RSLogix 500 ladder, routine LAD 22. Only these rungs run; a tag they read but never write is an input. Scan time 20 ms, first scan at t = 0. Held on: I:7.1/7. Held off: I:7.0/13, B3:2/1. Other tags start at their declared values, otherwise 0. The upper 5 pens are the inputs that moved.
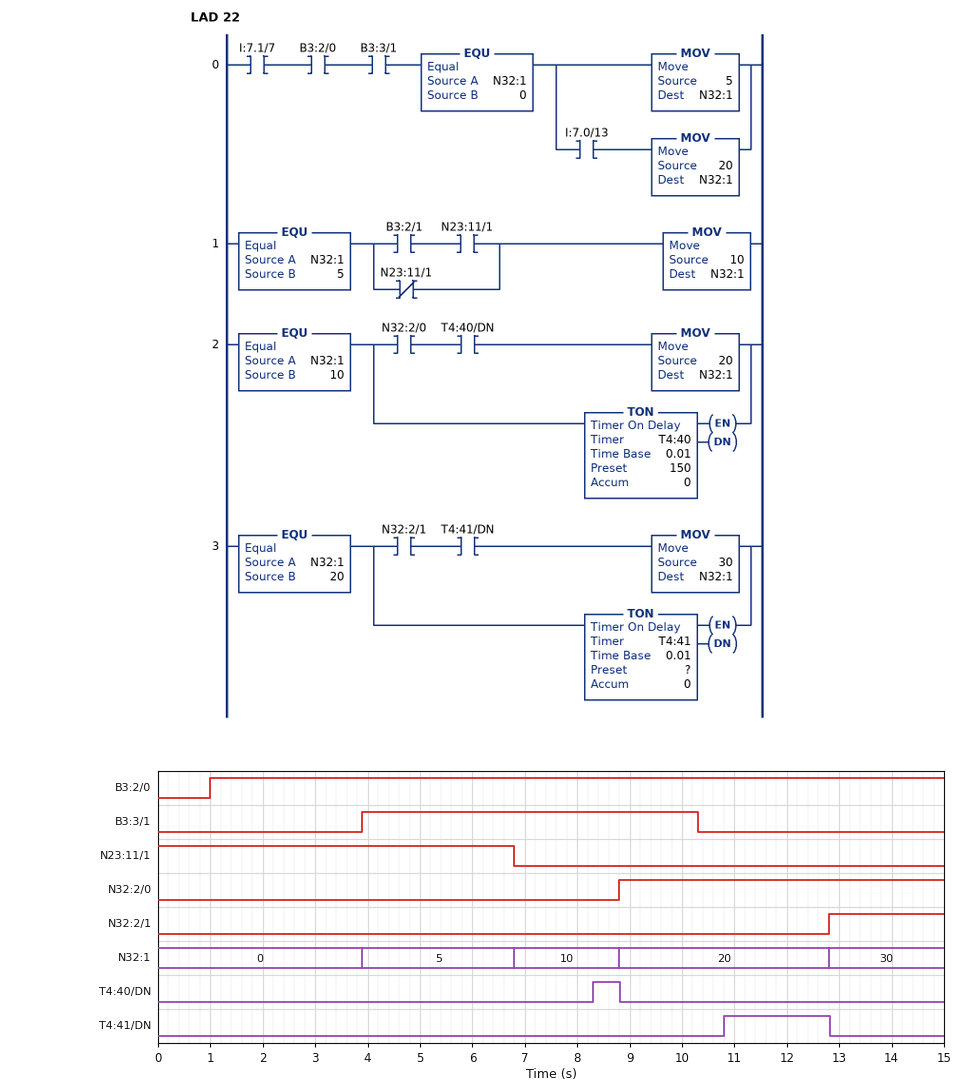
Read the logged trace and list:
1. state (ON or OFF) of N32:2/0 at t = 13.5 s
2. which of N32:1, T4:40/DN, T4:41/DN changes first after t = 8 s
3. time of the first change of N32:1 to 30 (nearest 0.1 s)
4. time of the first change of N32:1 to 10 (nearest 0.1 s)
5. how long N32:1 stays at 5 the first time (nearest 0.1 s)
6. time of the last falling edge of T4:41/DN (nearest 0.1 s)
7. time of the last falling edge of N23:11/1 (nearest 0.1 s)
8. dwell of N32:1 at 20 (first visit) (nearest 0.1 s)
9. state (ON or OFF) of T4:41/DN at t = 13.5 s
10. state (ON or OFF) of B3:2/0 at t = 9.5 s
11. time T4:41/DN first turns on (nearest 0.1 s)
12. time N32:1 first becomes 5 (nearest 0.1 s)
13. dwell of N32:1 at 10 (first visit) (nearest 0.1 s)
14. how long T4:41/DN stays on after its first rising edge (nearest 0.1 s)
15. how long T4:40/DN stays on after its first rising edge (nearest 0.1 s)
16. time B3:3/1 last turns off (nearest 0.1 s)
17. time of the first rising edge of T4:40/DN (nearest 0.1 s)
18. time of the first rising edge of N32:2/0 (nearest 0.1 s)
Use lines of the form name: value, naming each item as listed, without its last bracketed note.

state (ON or OFF) of N32:2/0 at t = 13.5 s: ON
which of N32:1, T4:40/DN, T4:41/DN changes first after t = 8 s: T4:40/DN
time of the first change of N32:1 to 30: 12.8 s
time of the first change of N32:1 to 10: 6.8 s
how long N32:1 stays at 5 the first time: 2.9 s
time of the last falling edge of T4:41/DN: 12.8 s
time of the last falling edge of N23:11/1: 6.8 s
dwell of N32:1 at 20 (first visit): 4.0 s
state (ON or OFF) of T4:41/DN at t = 13.5 s: OFF
state (ON or OFF) of B3:2/0 at t = 9.5 s: ON
time T4:41/DN first turns on: 10.8 s
time N32:1 first becomes 5: 3.9 s
dwell of N32:1 at 10 (first visit): 2.0 s
how long T4:41/DN stays on after its first rising edge: 2.0 s
how long T4:40/DN stays on after its first rising edge: 0.5 s
time B3:3/1 last turns off: 10.3 s
time of the first rising edge of T4:40/DN: 8.3 s
time of the first rising edge of N32:2/0: 8.8 s
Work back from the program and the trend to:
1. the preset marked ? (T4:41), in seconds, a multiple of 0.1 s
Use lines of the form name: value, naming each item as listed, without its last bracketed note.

the preset marked ? (T4:41), in seconds, a multiple of 0.1 s: 2.0 s
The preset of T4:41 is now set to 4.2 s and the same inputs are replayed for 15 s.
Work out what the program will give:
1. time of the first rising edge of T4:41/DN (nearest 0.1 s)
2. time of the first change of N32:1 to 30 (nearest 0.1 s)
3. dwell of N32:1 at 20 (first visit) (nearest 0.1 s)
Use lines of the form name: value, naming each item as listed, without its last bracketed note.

time of the first rising edge of T4:41/DN: 13.0 s
time of the first change of N32:1 to 30: 13.0 s
dwell of N32:1 at 20 (first visit): 4.2 s
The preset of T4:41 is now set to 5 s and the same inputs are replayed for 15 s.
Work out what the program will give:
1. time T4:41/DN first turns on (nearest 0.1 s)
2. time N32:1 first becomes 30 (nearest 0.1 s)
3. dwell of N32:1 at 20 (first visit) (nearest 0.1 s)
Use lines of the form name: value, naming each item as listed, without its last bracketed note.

time T4:41/DN first turns on: 13.8 s
time N32:1 first becomes 30: 13.8 s
dwell of N32:1 at 20 (first visit): 5.0 s
